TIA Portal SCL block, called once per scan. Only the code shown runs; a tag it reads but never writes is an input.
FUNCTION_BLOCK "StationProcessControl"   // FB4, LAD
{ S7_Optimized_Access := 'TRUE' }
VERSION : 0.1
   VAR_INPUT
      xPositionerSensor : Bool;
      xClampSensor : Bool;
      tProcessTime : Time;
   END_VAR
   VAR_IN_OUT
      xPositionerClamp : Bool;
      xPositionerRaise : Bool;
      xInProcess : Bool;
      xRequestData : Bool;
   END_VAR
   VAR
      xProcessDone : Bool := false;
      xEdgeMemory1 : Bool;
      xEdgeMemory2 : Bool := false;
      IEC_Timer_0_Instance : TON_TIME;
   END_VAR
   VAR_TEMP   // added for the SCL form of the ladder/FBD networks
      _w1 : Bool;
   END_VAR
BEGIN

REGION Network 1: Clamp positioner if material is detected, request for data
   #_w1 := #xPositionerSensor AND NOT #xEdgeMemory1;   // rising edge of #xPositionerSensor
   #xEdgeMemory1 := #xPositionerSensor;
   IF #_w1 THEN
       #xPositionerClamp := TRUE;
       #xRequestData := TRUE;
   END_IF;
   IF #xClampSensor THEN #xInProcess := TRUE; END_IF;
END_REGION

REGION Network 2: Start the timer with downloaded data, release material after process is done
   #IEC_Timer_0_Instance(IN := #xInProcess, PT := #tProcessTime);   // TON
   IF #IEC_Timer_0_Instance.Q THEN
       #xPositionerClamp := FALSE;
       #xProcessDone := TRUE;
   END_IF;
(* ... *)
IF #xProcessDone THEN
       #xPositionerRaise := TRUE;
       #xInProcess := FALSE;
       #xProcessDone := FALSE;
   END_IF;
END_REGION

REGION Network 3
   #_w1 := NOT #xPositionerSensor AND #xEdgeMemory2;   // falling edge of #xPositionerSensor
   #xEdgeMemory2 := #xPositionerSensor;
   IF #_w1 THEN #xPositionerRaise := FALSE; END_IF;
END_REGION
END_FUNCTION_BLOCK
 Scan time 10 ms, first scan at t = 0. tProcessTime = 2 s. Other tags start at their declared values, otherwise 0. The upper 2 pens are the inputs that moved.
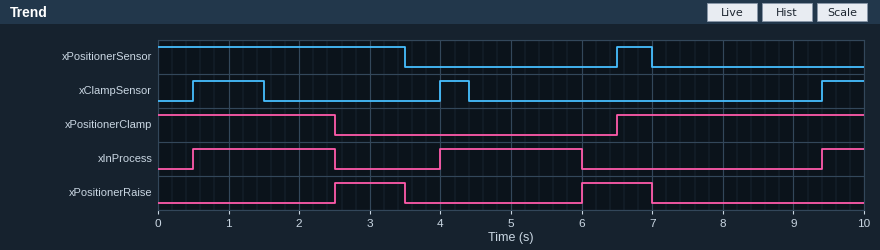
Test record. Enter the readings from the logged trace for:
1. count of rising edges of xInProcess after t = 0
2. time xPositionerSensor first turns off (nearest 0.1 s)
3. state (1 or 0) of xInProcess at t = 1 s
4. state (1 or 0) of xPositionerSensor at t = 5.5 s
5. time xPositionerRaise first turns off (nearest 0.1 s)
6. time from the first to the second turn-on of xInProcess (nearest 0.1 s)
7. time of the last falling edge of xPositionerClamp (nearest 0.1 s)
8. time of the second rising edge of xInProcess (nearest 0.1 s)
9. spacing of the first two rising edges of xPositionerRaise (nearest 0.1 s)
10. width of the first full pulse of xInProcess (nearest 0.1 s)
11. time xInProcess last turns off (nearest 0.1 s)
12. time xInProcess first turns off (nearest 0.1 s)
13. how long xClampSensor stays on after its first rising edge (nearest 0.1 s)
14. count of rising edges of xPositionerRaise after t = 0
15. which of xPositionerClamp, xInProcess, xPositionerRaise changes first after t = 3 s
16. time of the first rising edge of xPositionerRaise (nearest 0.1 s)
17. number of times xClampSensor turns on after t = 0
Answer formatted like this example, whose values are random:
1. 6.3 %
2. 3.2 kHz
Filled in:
1. 3
2. 3.5 s
3. 1
4. 0
5. 3.5 s
6. 3.5 s
7. 2.5 s
8. 4.0 s
9. 3.5 s
10. 2.0 s
11. 6.0 s
12. 2.5 s
13. 1.0 s
14. 2
15. xPositionerRaise
16. 2.5 s
17. 3
